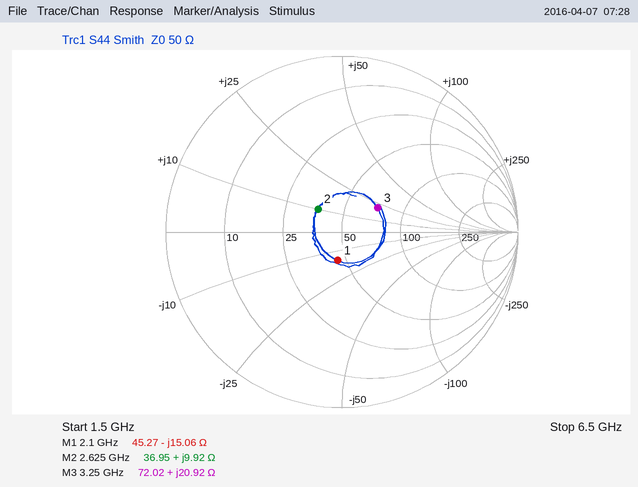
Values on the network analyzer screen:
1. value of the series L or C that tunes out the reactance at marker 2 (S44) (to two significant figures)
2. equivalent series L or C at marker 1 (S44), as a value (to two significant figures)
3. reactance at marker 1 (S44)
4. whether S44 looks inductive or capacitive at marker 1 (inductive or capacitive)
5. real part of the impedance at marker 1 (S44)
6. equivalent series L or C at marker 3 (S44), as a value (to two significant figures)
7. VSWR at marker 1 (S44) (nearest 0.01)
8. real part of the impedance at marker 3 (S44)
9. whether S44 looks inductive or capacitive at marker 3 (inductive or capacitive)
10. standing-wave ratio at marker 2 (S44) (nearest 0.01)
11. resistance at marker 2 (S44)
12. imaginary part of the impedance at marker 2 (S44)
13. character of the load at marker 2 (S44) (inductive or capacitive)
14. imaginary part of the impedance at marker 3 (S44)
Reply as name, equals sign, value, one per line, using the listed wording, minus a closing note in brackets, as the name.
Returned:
value of the series L or C that tunes out the reactance at marker 2 (S44) = 6.1 pF
equivalent series L or C at marker 1 (S44), as a value = 5.0 pF
reactance at marker 1 = -15.06 Ω
whether S44 looks inductive or capacitive at marker 1 = capacitive
real part of the impedance at marker 1 = 45.27 Ω
equivalent series L or C at marker 3 (S44), as a value = 1.0 nH
VSWR at marker 1 (S44) = 1.39
real part of the impedance at marker 3 = 72.02 Ω
whether S44 looks inductive or capacitive at marker 3 = inductive
standing-wave ratio at marker 2 (S44) = 1.46
resistance at marker 2 = 36.95 Ω
imaginary part of the impedance at marker 2 = +9.92 Ω
character of the load at marker 2 (S44) = inductive
imaginary part of the impedance at marker 3 = +20.92 Ω
